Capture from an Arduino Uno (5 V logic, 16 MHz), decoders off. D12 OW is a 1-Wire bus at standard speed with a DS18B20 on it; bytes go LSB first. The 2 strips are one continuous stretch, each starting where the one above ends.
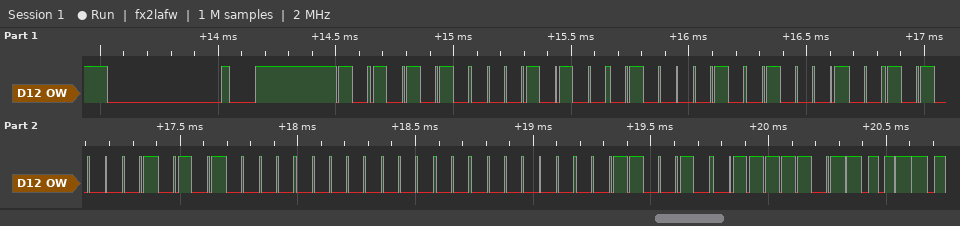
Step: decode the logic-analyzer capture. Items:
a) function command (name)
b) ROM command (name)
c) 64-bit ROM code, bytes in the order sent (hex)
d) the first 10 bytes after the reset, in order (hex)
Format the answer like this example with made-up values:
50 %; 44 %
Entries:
Read Scratchpad; Match ROM; 28 42 22 85 0A 00 00 4C; 55 28 42 22 85 0A 00 00 4C BE
